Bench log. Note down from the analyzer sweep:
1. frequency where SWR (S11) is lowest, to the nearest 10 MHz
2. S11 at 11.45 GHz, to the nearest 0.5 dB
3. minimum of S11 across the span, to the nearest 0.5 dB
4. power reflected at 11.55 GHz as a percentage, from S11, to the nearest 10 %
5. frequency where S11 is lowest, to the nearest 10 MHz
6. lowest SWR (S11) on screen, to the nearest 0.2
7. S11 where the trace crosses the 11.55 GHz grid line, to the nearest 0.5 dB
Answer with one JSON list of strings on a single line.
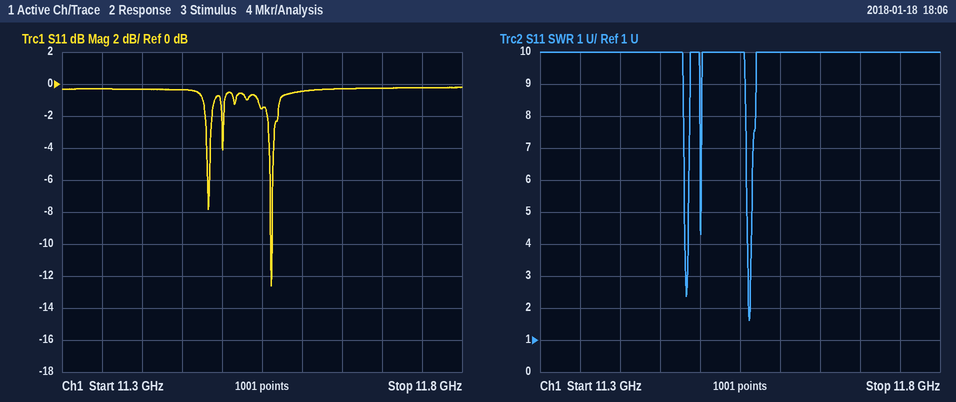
["11.56 GHz", "-0.5 dB", "-12.5 dB", "70 %", "11.56 GHz", "1.6", "-1.5 dB"]
